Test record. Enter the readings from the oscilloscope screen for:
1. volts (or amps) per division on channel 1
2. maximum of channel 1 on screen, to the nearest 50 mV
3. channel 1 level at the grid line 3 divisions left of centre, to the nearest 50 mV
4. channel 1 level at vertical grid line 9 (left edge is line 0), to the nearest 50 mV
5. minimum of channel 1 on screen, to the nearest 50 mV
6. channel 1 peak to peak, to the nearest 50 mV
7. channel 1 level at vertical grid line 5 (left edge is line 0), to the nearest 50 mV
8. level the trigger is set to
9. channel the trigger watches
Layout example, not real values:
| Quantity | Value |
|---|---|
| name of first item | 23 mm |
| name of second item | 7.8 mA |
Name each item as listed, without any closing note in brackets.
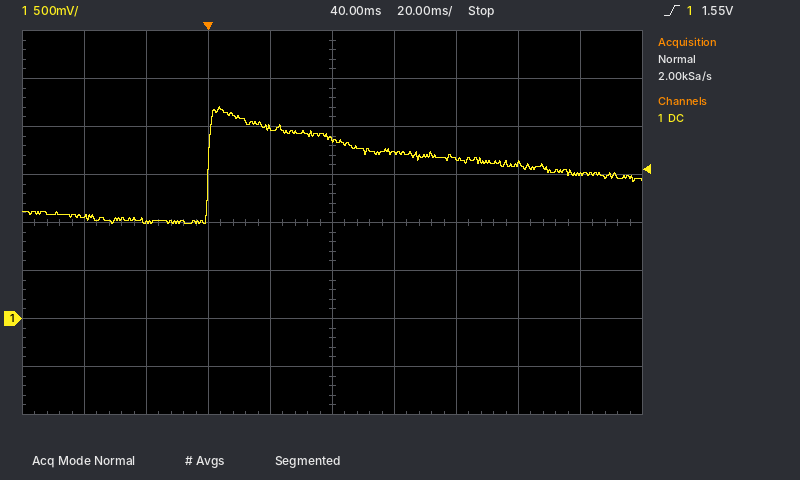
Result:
| Quantity | Value |
|---|---|
| volts (or amps) per division on channel 1 | 500 mV |
| maximum of channel 1 on screen, to the nearest 50 mV | 2.20 V |
| channel 1 level at the grid line 3 divisions left of centre, to the nearest 50 mV | 1.00 V |
| channel 1 level at vertical grid line 9 (left edge is line 0), to the nearest 50 mV | 1.50 V |
| minimum of channel 1 on screen, to the nearest 50 mV | 1.00 V |
| channel 1 peak to peak, to the nearest 50 mV | 1.20 V |
| channel 1 level at vertical grid line 5 (left edge is line 0), to the nearest 50 mV | 1.85 V |
| level the trigger is set to | 1.55 V |
| channel the trigger watches | channel 1 |
